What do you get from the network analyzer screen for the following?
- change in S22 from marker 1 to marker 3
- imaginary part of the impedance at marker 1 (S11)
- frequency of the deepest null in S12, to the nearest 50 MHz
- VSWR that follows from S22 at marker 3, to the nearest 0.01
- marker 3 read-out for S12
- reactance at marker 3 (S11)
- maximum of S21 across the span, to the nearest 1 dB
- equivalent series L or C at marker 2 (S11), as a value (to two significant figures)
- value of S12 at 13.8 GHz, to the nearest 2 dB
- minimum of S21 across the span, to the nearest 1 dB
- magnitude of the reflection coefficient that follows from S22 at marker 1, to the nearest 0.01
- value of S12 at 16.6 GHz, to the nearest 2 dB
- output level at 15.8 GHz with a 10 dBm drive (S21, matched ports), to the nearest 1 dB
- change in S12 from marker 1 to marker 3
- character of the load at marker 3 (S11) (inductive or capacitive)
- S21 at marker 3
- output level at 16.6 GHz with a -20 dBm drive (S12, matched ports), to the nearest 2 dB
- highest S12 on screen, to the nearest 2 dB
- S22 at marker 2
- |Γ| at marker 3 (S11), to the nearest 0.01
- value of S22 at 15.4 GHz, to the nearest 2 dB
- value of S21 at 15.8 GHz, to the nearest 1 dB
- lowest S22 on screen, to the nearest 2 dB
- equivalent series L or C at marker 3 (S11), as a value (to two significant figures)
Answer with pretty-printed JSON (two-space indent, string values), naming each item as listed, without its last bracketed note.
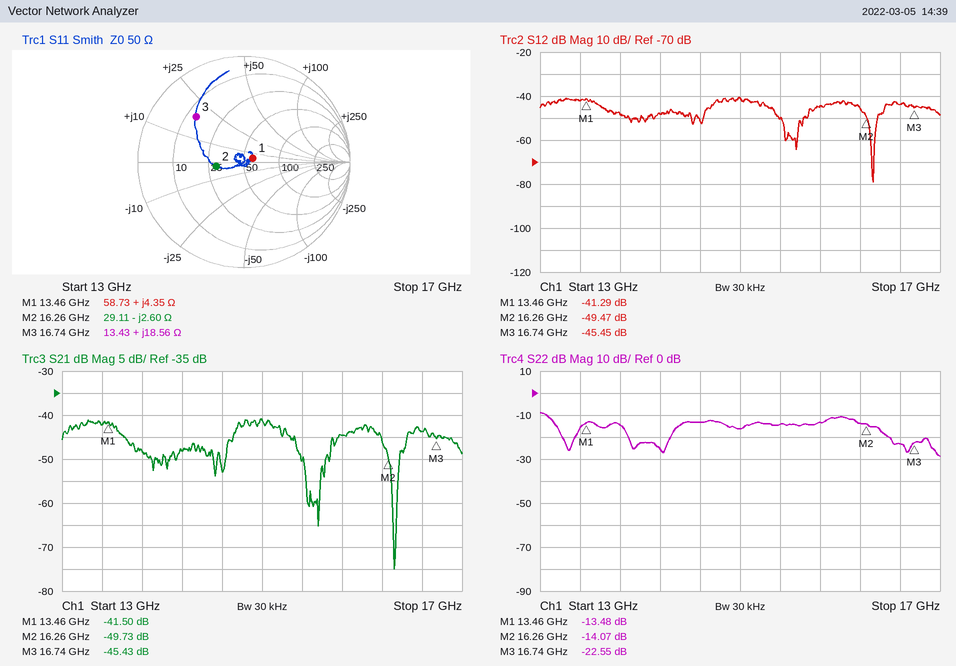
{
  "change in S22 from marker 1 to marker 3": "-9.07 dB",
  "imaginary part of the impedance at marker 1": "+4.35 Ω",
  "frequency of the deepest null in S12, to the nearest 50 MHz": "16.35 GHz",
  "VSWR that follows from S22 at marker 3, to the nearest 0.01": "1.16",
  "marker 3 read-out for S12": "-45.45 dB",
  "reactance at marker 3": "+18.56 Ω",
  "maximum of S21 across the span, to the nearest 1 dB": "-41 dB",
  "equivalent series L or C at marker 2 (S11), as a value": "3.8 pF",
  "value of S12 at 13.8 GHz, to the nearest 2 dB": "-48 dB",
  "minimum of S21 across the span, to the nearest 1 dB": "-75 dB",
  "magnitude of the reflection coefficient that follows from S22 at marker 1, to the nearest 0.01": "0.21",
  "value of S12 at 16.6 GHz, to the nearest 2 dB": "-44 dB",
  "output level at 15.8 GHz with a 10 dBm drive (S21, matched ports), to the nearest 1 dB": "-35 dBm",
  "change in S12 from marker 1 to marker 3": "-4.16 dB",
  "character of the load at marker 3 (S11)": "inductive",
  "S21 at marker 3": "-45.43 dB",
  "output level at 16.6 GHz with a -20 dBm drive (S12, matched ports), to the nearest 2 dB": "-64 dBm",
  "highest S12 on screen, to the nearest 2 dB": "-40 dB",
  "S22 at marker 2": "-14.07 dB",
  "|Γ| at marker 3 (S11), to the nearest 0.01": "0.62",
  "value of S22 at 15.4 GHz, to the nearest 2 dB": "-14 dB",
  "value of S21 at 15.8 GHz, to the nearest 1 dB": "-45 dB",
  "lowest S22 on screen, to the nearest 2 dB": "-28 dB",
  "equivalent series L or C at marker 3 (S11), as a value": "180 pH"
}
